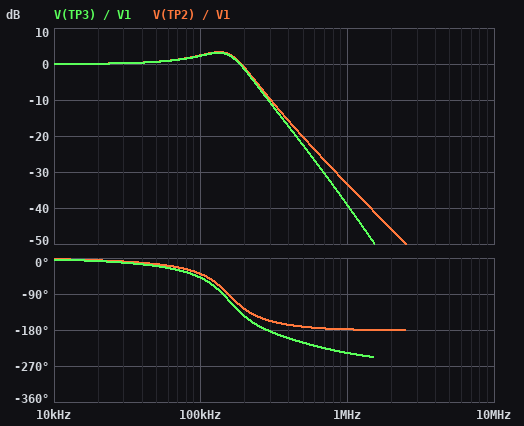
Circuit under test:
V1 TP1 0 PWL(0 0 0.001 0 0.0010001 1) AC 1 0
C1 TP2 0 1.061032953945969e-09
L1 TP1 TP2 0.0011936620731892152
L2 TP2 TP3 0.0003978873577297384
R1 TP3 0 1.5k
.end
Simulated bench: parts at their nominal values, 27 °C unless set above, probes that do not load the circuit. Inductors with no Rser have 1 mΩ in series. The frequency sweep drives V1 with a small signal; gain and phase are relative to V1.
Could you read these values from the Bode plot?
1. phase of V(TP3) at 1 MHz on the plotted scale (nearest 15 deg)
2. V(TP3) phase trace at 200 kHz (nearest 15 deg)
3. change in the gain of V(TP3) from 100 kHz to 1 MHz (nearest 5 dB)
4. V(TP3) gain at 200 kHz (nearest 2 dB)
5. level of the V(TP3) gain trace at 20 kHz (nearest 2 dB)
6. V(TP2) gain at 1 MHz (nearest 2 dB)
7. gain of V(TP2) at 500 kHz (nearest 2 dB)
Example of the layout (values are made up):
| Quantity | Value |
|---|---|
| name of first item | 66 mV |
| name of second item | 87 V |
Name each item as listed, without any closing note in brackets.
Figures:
| Quantity | Value |
|---|---|
| phase of V(TP3) at 1 MHz on the plotted scale | -240 deg |
| V(TP3) phase trace at 200 kHz | -150 deg |
| change in the gain of V(TP3) from 100 kHz to 1 MHz | -40 dB |
| V(TP3) gain at 200 kHz | -2 dB |
| level of the V(TP3) gain trace at 20 kHz | 0 dB |
| V(TP2) gain at 1 MHz | -34 dB |
| gain of V(TP2) at 500 kHz | -20 dB |
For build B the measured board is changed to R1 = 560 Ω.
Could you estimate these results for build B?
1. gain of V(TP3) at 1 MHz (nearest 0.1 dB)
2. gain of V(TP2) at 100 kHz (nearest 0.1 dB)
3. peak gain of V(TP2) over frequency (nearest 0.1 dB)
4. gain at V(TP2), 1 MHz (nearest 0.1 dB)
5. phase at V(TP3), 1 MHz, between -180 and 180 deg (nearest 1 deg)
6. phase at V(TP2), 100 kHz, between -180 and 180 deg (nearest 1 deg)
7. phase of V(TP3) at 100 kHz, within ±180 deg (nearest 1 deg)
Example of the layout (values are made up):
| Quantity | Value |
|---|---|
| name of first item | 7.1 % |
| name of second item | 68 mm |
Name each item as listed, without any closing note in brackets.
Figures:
| Quantity | Value |
|---|---|
| gain of V(TP3) at 1 MHz | -46.5 dB |
| gain of V(TP2) at 100 kHz | -3.5 dB |
| peak gain of V(TP2) over frequency | 0 dB |
| gain at V(TP2), 1 MHz | -33.3 dB |
| phase at V(TP3), 1 MHz, between -180 and 180 deg | 103 deg |
| phase at V(TP2), 100 kHz, between -180 and 180 deg | -48 deg |
| phase of V(TP3) at 100 kHz, within ±180 deg | -72 deg |
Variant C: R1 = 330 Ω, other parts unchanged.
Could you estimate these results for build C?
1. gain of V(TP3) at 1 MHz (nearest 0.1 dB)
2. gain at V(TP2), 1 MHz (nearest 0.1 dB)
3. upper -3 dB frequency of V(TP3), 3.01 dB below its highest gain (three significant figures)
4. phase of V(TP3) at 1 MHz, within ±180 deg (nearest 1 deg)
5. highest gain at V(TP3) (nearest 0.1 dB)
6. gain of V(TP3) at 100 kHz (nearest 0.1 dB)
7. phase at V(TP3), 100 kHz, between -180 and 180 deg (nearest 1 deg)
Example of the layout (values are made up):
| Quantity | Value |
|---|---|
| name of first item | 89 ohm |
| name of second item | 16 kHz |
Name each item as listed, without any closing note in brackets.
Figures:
| Quantity | Value |
|---|---|
| gain of V(TP3) at 1 MHz | -50.9 dB |
| gain at V(TP2), 1 MHz | -33.3 dB |
| upper -3 dB frequency of V(TP3), 3.01 dB below its highest gain | 35.5 kHz |
| phase of V(TP3) at 1 MHz, within ±180 deg | 98 deg |
| highest gain at V(TP3) | 0 dB |
| gain of V(TP3) at 100 kHz | -8.6 dB |
| phase at V(TP3), 100 kHz, between -180 and 180 deg | -79 deg |
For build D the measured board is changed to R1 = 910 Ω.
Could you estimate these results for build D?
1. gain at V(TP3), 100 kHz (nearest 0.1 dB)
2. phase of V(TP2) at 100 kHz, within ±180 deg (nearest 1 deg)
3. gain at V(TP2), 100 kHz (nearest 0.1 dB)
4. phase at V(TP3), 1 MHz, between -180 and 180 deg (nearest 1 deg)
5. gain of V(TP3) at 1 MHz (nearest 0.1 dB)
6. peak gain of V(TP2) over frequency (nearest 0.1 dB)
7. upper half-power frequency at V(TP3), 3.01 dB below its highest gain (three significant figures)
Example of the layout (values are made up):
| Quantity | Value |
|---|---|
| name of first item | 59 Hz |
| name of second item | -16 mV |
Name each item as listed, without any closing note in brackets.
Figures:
| Quantity | Value |
|---|---|
| gain at V(TP3), 100 kHz | -0.7 dB |
| phase of V(TP2) at 100 kHz, within ±180 deg | -47 deg |
| gain at V(TP2), 100 kHz | -0.4 dB |
| phase at V(TP3), 1 MHz, between -180 and 180 deg | 111 deg |
| gain of V(TP3) at 1 MHz | -42.6 dB |
| peak gain of V(TP2) over frequency | 0 dB |
| upper half-power frequency at V(TP3), 3.01 dB below its highest gain | 192 kHz |
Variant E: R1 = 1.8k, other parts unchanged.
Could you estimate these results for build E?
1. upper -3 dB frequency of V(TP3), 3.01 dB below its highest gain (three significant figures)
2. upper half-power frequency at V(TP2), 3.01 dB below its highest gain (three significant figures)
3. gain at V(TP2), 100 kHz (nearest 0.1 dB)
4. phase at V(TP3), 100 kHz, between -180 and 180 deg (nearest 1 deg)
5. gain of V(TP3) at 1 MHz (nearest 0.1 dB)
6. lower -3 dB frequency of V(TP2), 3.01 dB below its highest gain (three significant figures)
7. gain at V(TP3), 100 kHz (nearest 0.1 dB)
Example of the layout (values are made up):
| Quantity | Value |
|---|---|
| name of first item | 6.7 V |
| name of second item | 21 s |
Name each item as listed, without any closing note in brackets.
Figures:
| Quantity | Value |
|---|---|
| upper -3 dB frequency of V(TP3), 3.01 dB below its highest gain | 177 kHz |
| upper half-power frequency at V(TP2), 3.01 dB below its highest gain | 178 kHz |
| gain at V(TP2), 100 kHz | 3.2 dB |
| phase at V(TP3), 100 kHz, between -180 and 180 deg | -44 deg |
| gain of V(TP3) at 1 MHz | -38.1 dB |
| lower -3 dB frequency of V(TP2), 3.01 dB below its highest gain | 74.6 kHz |
| gain at V(TP3), 100 kHz | 3.1 dB |
